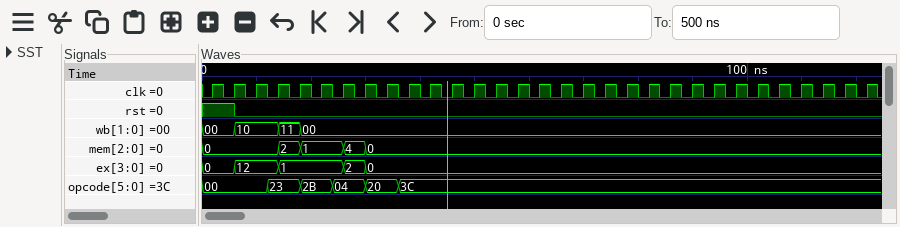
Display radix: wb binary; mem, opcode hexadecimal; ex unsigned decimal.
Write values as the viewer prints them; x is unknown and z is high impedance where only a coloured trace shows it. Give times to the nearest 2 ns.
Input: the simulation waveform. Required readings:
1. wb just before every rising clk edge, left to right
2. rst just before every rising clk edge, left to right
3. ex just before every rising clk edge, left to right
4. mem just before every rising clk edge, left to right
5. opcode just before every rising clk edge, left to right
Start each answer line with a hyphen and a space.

- 00, 00, 10, 10, 11, 00, 00, 00, 00, 00, 00, 00, 00, 00, 00, 00, 00, 00, 00, 00, 00, 00, 00, 00, 00, 00, 00, 00, 00, 00, 00
- 1 1 0 0 0 0 0 0 0 0 0 0 0 0 0 0 0 0 0 0 0 0 0 0 0 0 0 0 0 0 0
- 0, 0, 12, 12, 1, 1, 1, 2, 0, 0, 0, 0, 0, 0, 0, 0, 0, 0, 0, 0, 0, 0, 0, 0, 0, 0, 0, 0, 0, 0, 0
- 0, 0, 0, 0, 2, 1, 1, 4, 0, 0, 0, 0, 0, 0, 0, 0, 0, 0, 0, 0, 0, 0, 0, 0, 0, 0, 0, 0, 0, 0, 0
- 00, 00, 00, 23, 23, 2B, 04, 04, 20, 3C, 3C, 3C, 3C, 3C, 3C, 3C, 3C, 3C, 3C, 3C, 3C, 3C, 3C, 3C, 3C, 3C, 3C, 3C, 3C, 3C, 3C
